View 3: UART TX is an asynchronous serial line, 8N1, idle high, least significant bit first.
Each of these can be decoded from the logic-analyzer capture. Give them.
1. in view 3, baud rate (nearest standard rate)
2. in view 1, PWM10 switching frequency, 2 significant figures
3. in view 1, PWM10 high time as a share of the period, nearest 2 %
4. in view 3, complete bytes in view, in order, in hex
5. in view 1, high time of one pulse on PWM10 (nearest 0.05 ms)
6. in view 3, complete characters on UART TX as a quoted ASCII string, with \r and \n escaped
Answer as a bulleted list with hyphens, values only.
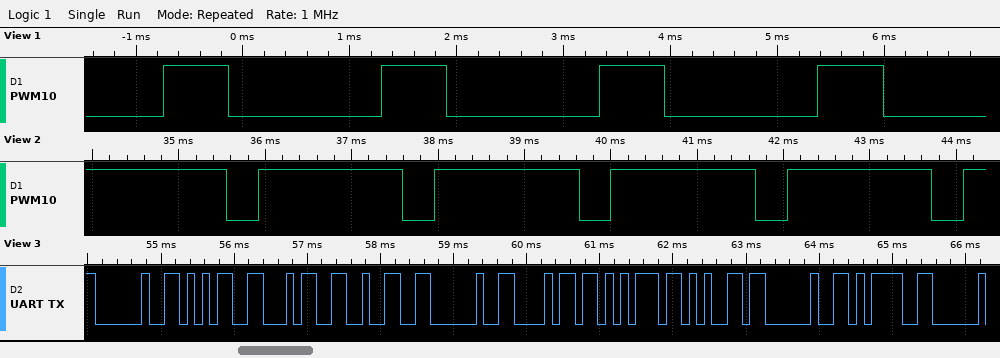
- 9600 baud
- 490 Hz
- 30 %
- 0x20 0x35 0x34 0x32 0x20 0x68 0x75 0x65 0x20 0x3D
- 0.60 ms
- " 542 hue ="
